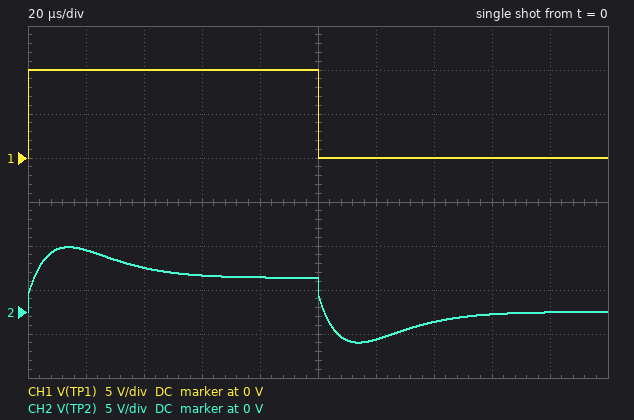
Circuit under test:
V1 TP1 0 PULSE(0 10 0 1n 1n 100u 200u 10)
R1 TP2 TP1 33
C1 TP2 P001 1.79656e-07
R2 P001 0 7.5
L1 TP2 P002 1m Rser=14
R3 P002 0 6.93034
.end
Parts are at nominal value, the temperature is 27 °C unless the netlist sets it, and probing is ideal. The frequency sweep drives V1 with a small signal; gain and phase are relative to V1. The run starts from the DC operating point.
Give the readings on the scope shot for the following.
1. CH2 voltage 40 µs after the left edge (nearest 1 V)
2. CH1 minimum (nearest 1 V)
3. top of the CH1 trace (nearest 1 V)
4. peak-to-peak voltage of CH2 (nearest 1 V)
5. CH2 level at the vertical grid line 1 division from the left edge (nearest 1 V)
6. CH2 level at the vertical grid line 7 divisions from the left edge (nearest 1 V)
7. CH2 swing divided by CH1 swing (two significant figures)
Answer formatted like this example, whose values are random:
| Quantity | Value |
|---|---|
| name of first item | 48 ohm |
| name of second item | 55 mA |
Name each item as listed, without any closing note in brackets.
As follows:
| Quantity | Value |
|---|---|
| CH2 voltage 40 µs after the left edge | 5 V |
| CH1 minimum | 0 V |
| top of the CH1 trace | 10 V |
| peak-to-peak voltage of CH2 | 11 V |
| CH2 level at the vertical grid line 1 division from the left edge | 7 V |
| CH2 level at the vertical grid line 7 divisions from the left edge | -1 V |
| CH2 swing divided by CH1 swing | 1.1 |
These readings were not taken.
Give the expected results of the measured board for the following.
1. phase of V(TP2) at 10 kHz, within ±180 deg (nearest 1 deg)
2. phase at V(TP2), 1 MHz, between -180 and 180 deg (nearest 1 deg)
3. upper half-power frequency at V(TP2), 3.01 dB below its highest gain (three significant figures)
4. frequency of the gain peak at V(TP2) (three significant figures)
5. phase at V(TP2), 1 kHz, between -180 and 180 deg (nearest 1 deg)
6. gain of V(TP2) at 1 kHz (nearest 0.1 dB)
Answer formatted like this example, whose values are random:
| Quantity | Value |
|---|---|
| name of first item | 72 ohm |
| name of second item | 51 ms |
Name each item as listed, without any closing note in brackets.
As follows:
| Quantity | Value |
|---|---|
| phase of V(TP2) at 10 kHz, within ±180 deg | 5 deg |
| phase at V(TP2), 1 MHz, between -180 and 180 deg | -5 deg |
| upper half-power frequency at V(TP2), 3.01 dB below its highest gain | 32.3 kHz |
| frequency of the gain peak at V(TP2) | 13.1 kHz |
| phase at V(TP2), 1 kHz, between -180 and 180 deg | 9 deg |
| gain of V(TP2) at 1 kHz | -7.9 dB |
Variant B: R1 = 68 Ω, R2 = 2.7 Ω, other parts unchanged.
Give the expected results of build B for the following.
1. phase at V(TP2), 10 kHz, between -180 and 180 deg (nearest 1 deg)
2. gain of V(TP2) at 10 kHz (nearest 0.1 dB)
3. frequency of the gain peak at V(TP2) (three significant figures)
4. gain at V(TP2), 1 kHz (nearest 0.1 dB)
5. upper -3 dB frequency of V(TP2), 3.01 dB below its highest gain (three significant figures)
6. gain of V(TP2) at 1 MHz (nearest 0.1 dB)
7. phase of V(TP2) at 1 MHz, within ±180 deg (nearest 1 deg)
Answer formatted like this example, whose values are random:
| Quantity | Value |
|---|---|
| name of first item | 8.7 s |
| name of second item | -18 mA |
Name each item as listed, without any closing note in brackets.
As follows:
| Quantity | Value |
|---|---|
| phase at V(TP2), 10 kHz, between -180 and 180 deg | 9 deg |
| gain of V(TP2) at 10 kHz | -2.7 dB |
| frequency of the gain peak at V(TP2) | 13.0 kHz |
| gain at V(TP2), 1 kHz | -12.2 dB |
| upper -3 dB frequency of V(TP2), 3.01 dB below its highest gain | 23.3 kHz |
| gain of V(TP2) at 1 MHz | -27.9 dB |
| phase of V(TP2) at 1 MHz, within ±180 deg | -17 deg |
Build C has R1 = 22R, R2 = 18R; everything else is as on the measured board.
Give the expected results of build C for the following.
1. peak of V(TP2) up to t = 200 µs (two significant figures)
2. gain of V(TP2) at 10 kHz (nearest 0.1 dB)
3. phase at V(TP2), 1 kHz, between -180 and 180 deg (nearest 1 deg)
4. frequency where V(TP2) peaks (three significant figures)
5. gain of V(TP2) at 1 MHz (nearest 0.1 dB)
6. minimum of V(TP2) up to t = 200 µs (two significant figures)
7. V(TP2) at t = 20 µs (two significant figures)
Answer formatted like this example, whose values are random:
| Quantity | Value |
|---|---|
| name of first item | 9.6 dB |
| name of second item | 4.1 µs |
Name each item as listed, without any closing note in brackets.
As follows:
| Quantity | Value |
|---|---|
| peak of V(TP2) up to t = 200 µs | 7.8 V |
| gain of V(TP2) at 10 kHz | -1.3 dB |
| phase at V(TP2), 1 kHz, between -180 and 180 deg | 8 deg |
| frequency where V(TP2) peaks | 12.1 kHz |
| gain of V(TP2) at 1 MHz | -6.9 dB |
| minimum of V(TP2) up to t = 200 µs | -2.9 V |
| V(TP2) at t = 20 µs | 7.5 V |
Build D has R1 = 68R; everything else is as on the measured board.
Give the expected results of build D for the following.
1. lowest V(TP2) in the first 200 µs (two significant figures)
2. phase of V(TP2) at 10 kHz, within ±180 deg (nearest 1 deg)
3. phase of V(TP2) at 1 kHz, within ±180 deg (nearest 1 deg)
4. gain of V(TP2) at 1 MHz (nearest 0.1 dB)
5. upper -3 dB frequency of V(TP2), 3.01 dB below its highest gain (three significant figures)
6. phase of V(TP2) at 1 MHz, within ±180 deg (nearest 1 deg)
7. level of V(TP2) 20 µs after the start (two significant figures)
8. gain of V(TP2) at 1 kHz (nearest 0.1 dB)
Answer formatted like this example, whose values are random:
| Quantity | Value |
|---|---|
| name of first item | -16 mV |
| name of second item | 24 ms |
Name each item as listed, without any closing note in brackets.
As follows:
| Quantity | Value |
|---|---|
| lowest V(TP2) in the first 200 µs | -3.2 V |
| phase of V(TP2) at 10 kHz, within ±180 deg | 9 deg |
| phase of V(TP2) at 1 kHz, within ±180 deg | 12 deg |
| gain of V(TP2) at 1 MHz | -20.0 dB |
| upper -3 dB frequency of V(TP2), 3.01 dB below its highest gain | 23.0 kHz |
| phase of V(TP2) at 1 MHz, within ±180 deg | -6 deg |
| level of V(TP2) 20 µs after the start | 5.4 V |
| gain of V(TP2) at 1 kHz | -12.2 dB |
